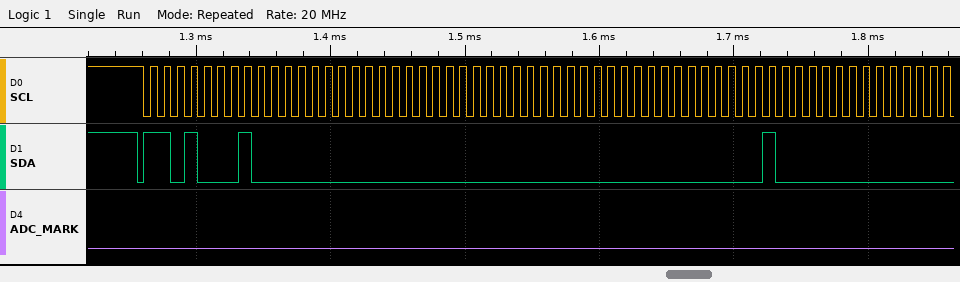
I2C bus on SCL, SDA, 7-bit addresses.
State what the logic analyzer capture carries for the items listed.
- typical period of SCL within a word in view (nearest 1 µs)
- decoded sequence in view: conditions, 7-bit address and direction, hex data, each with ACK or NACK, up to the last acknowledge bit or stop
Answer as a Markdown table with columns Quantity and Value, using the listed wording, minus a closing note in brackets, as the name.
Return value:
| Quantity | Value |
|---|---|
| typical period of SCL within a word in view | 10 µs |
| decoded sequence in view: conditions, 7-bit address and direction, hex data, each with ACK or NACK, up to the last acknowledge bit or stop | start, address 68 read ACK, 00 ACK, 00 ACK, 00 ACK, 00 ACK, 40 ACK |
